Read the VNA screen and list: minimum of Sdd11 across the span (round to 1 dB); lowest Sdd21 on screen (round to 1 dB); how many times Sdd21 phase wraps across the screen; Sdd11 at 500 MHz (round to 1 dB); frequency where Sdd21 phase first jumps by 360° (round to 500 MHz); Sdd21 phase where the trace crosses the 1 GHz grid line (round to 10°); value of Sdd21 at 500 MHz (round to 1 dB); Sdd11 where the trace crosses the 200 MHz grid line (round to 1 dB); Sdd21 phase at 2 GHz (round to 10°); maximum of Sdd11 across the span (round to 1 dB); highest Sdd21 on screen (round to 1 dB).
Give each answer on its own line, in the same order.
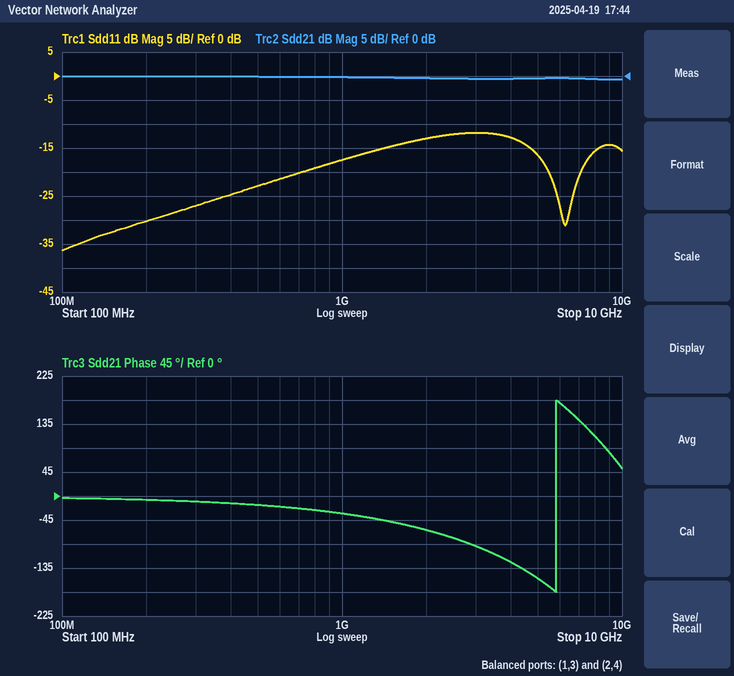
-36 dB
-1 dB
1
-23 dB
6.0 GHz
-30°
0 dB
-30 dB
-60°
-12 dB
0 dB
